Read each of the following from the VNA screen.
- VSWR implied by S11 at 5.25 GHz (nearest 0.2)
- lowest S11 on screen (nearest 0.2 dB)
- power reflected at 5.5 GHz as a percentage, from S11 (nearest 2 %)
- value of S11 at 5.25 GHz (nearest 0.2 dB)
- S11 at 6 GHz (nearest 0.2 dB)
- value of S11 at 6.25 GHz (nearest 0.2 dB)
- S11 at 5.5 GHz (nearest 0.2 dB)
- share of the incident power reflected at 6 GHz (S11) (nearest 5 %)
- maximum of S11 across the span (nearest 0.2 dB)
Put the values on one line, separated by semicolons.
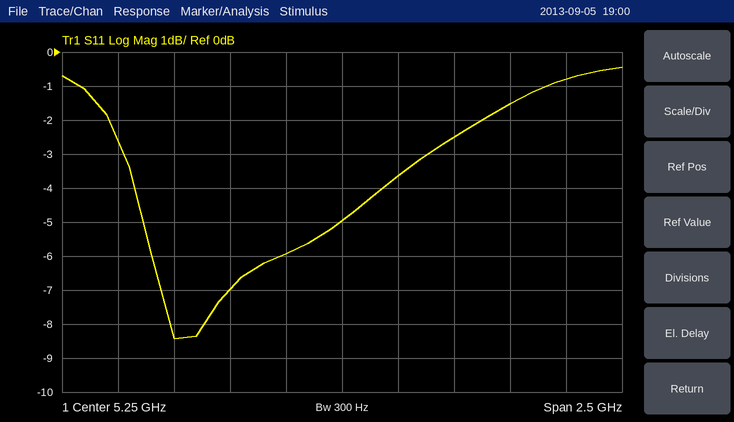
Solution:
3.6; -8.4 dB; 44 %; -5.0 dB; -1.6 dB; -0.8 dB; -3.6 dB; 70 %; -0.4 dB
